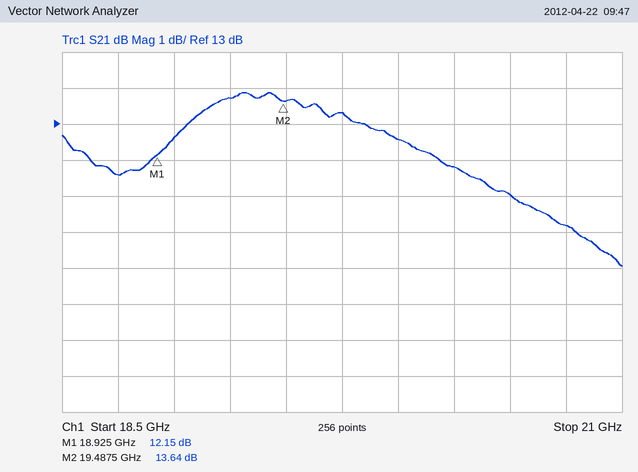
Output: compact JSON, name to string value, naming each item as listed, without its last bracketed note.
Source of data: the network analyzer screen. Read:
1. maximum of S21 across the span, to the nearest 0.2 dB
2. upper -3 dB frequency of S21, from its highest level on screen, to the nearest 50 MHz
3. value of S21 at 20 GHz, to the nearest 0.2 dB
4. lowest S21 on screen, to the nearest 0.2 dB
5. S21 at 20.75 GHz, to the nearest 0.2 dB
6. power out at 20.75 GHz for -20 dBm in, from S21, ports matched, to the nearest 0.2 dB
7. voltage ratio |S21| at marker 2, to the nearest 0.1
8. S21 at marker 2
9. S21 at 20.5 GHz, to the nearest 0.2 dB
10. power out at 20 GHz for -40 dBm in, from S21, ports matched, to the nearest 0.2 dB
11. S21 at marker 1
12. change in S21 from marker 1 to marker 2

{"maximum of S21 across the span, to the nearest 0.2 dB": "13.8 dB", "upper -3 dB frequency of S21, from its highest level on screen, to the nearest 50 MHz": "20.55 GHz", "value of S21 at 20 GHz, to the nearest 0.2 dB": "12.6 dB", "lowest S21 on screen, to the nearest 0.2 dB": "9.0 dB", "S21 at 20.75 GHz, to the nearest 0.2 dB": "10.2 dB", "power out at 20.75 GHz for -20 dBm in, from S21, ports matched, to the nearest 0.2 dB": "-9.8 dBm", "voltage ratio |S21| at marker 2, to the nearest 0.1": "4.8", "S21 at marker 2": "13.64 dB", "S21 at 20.5 GHz, to the nearest 0.2 dB": "11.0 dB", "power out at 20 GHz for -40 dBm in, from S21, ports matched, to the nearest 0.2 dB": "-27.4 dBm", "S21 at marker 1": "12.15 dB", "change in S21 from marker 1 to marker 2": "1.49 dB"}
